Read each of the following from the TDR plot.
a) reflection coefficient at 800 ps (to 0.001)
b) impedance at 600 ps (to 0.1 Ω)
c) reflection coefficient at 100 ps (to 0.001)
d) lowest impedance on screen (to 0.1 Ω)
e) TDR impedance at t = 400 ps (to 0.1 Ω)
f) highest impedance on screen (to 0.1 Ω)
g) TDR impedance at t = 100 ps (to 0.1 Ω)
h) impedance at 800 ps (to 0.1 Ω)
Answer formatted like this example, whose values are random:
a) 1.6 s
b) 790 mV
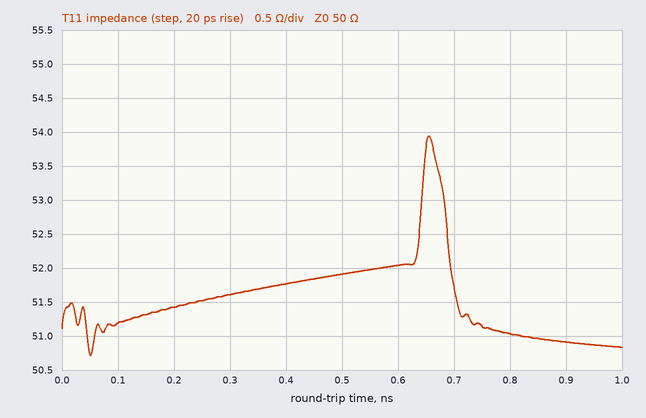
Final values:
a) +0.010
b) 52.0 Ω
c) +0.012
d) 50.7 Ω
e) 51.8 Ω
f) 53.9 Ω
g) 51.2 Ω
h) 51.0 Ω
